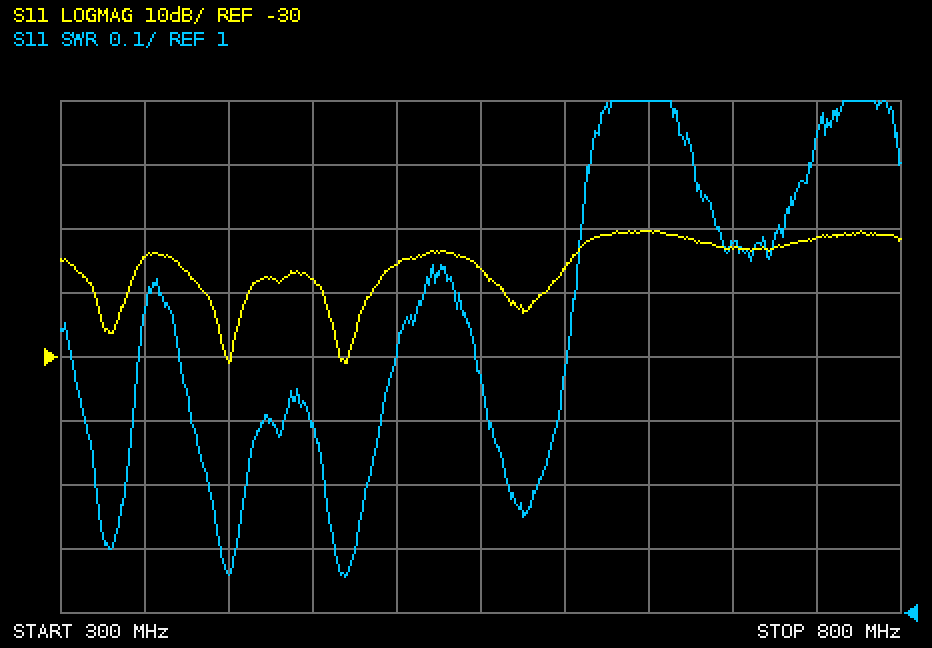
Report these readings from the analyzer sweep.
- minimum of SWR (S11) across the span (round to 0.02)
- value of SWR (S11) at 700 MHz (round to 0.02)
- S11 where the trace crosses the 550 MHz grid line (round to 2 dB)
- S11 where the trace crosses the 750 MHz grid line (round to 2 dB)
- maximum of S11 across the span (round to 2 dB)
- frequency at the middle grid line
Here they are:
1.06
1.58
-16 dB
-12 dB
-10 dB
550 MHz
